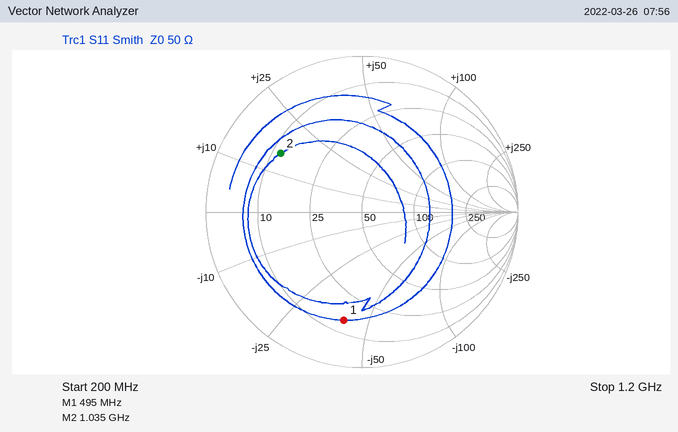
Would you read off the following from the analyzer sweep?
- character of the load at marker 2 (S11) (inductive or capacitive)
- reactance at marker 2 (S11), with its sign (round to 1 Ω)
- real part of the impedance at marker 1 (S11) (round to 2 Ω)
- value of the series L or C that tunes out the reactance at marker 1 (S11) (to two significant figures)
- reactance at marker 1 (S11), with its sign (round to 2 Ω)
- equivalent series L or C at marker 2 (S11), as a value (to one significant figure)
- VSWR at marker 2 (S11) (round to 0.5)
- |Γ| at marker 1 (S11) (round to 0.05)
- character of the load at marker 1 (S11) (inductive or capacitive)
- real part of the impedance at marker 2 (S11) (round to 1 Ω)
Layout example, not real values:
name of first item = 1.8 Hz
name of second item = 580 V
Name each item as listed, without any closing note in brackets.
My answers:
character of the load at marker 2 (S11) = inductive
reactance at marker 2 (S11), with its sign = +15 Ω
real part of the impedance at marker 1 (S11) = 14 Ω
value of the series L or C that tunes out the reactance at marker 1 (S11) = 13 nH
reactance at marker 1 (S11), with its sign = -40 Ω
equivalent series L or C at marker 2 (S11), as a value = 2 nH
VSWR at marker 2 (S11) = 4.5
|Γ| at marker 1 (S11) = 0.70
character of the load at marker 1 (S11) = capacitive
real part of the impedance at marker 2 (S11) = 12 Ω
